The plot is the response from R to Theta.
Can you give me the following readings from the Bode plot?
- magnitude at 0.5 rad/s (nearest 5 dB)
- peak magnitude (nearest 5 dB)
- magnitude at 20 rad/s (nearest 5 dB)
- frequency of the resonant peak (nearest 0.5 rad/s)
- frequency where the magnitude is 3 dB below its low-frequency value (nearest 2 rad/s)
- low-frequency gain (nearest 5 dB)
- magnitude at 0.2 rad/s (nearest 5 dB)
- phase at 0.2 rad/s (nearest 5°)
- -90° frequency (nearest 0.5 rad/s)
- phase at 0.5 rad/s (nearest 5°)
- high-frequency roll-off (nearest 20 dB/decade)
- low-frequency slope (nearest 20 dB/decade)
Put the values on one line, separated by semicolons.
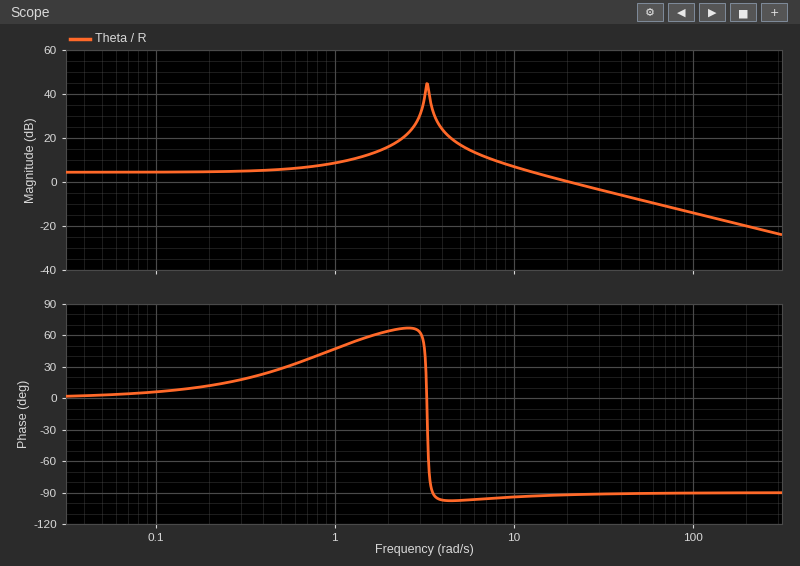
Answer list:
5 dB; 45 dB; 0 dB; 3.5 rad/s; 18 rad/s; 5 dB; 5 dB; 10°; 3.5 rad/s; 30°; -20 dB/decade; 0 dB/decade
